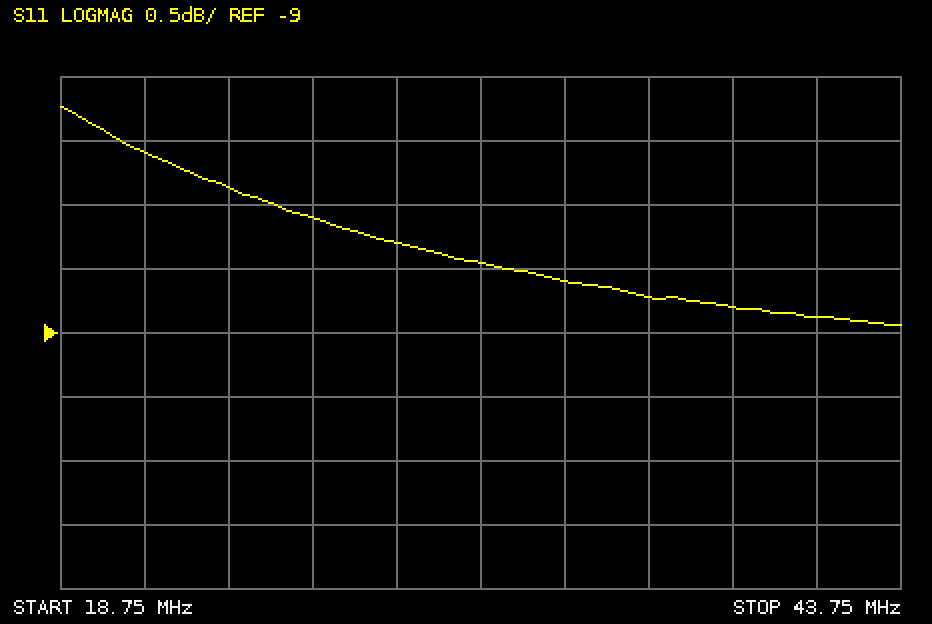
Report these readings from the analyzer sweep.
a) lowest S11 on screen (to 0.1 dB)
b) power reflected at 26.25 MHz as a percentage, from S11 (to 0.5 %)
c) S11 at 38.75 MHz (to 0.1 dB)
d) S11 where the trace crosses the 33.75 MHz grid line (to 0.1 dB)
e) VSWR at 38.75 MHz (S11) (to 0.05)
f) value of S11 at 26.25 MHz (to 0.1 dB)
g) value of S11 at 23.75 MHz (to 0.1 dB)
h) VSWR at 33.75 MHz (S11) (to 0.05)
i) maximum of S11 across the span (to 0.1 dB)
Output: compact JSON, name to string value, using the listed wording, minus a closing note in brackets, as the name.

{"lowest S11 on screen": "-8.9 dB", "power reflected at 26.25 MHz as a percentage, from S11": "15.5 %", "S11 at 38.75 MHz": "-8.8 dB", "S11 where the trace crosses the 33.75 MHz grid line": "-8.6 dB", "VSWR at 38.75 MHz (S11)": "2.15", "value of S11 at 26.25 MHz": "-8.1 dB", "value of S11 at 23.75 MHz": "-7.9 dB", "VSWR at 33.75 MHz (S11)": "2.20", "maximum of S11 across the span": "-7.2 dB"}
